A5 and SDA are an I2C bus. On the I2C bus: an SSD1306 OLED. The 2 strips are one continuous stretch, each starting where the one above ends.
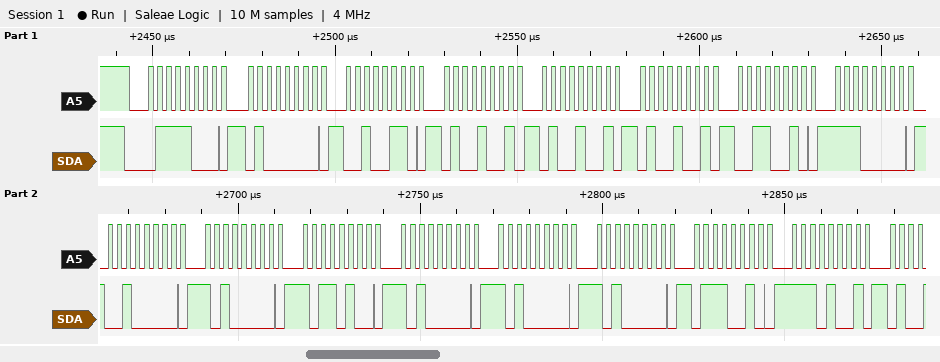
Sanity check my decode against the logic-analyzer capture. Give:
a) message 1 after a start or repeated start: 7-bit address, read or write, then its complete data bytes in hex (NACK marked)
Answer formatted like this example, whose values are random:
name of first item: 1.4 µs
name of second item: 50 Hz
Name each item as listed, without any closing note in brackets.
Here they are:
message 1 after a start or repeated start: 7-bit address, read or write, then its complete data bytes in hex: 0x3C write: 40 26 49 49 49 32 E0 20 A0 B4 A0 A0 A0 72 E9
